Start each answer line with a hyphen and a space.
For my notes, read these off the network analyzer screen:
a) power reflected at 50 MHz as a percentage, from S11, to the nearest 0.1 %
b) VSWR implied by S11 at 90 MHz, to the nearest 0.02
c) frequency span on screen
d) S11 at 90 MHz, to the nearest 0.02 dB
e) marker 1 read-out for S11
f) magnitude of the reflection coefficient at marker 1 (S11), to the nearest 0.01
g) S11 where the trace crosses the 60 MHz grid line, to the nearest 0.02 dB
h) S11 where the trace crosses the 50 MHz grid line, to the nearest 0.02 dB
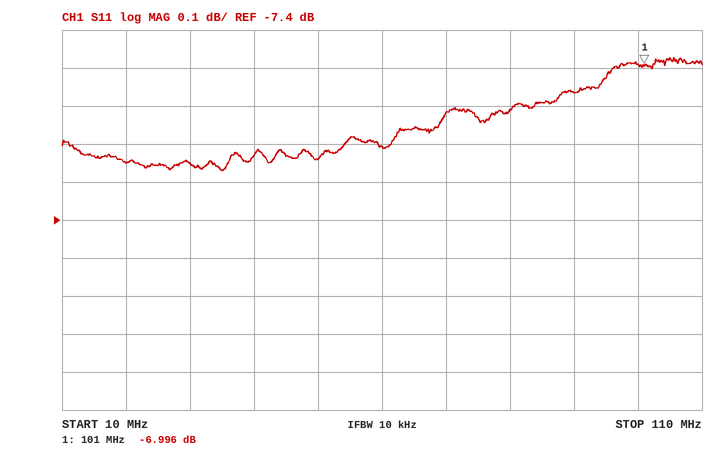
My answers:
- 18.9 %
- 2.60
- 100 MHz
- -7.06 dB
- -6.996 dB
- 0.45
- -7.20 dB
- -7.24 dB
